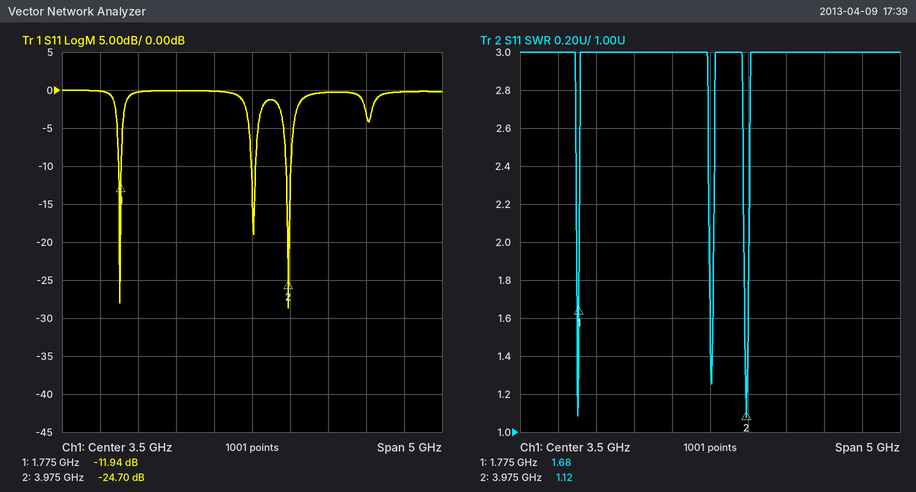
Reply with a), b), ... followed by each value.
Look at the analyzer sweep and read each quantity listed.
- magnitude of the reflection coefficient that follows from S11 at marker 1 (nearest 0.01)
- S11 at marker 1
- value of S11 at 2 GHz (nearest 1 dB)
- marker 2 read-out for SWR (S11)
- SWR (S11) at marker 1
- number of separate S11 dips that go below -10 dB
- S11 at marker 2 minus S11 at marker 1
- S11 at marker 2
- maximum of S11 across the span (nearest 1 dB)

a) 0.25
b) -11.94 dB
c) 0 dB
d) 1.12
e) 1.68
f) 3
g) -12.76 dB
h) -24.70 dB
i) 0 dB
